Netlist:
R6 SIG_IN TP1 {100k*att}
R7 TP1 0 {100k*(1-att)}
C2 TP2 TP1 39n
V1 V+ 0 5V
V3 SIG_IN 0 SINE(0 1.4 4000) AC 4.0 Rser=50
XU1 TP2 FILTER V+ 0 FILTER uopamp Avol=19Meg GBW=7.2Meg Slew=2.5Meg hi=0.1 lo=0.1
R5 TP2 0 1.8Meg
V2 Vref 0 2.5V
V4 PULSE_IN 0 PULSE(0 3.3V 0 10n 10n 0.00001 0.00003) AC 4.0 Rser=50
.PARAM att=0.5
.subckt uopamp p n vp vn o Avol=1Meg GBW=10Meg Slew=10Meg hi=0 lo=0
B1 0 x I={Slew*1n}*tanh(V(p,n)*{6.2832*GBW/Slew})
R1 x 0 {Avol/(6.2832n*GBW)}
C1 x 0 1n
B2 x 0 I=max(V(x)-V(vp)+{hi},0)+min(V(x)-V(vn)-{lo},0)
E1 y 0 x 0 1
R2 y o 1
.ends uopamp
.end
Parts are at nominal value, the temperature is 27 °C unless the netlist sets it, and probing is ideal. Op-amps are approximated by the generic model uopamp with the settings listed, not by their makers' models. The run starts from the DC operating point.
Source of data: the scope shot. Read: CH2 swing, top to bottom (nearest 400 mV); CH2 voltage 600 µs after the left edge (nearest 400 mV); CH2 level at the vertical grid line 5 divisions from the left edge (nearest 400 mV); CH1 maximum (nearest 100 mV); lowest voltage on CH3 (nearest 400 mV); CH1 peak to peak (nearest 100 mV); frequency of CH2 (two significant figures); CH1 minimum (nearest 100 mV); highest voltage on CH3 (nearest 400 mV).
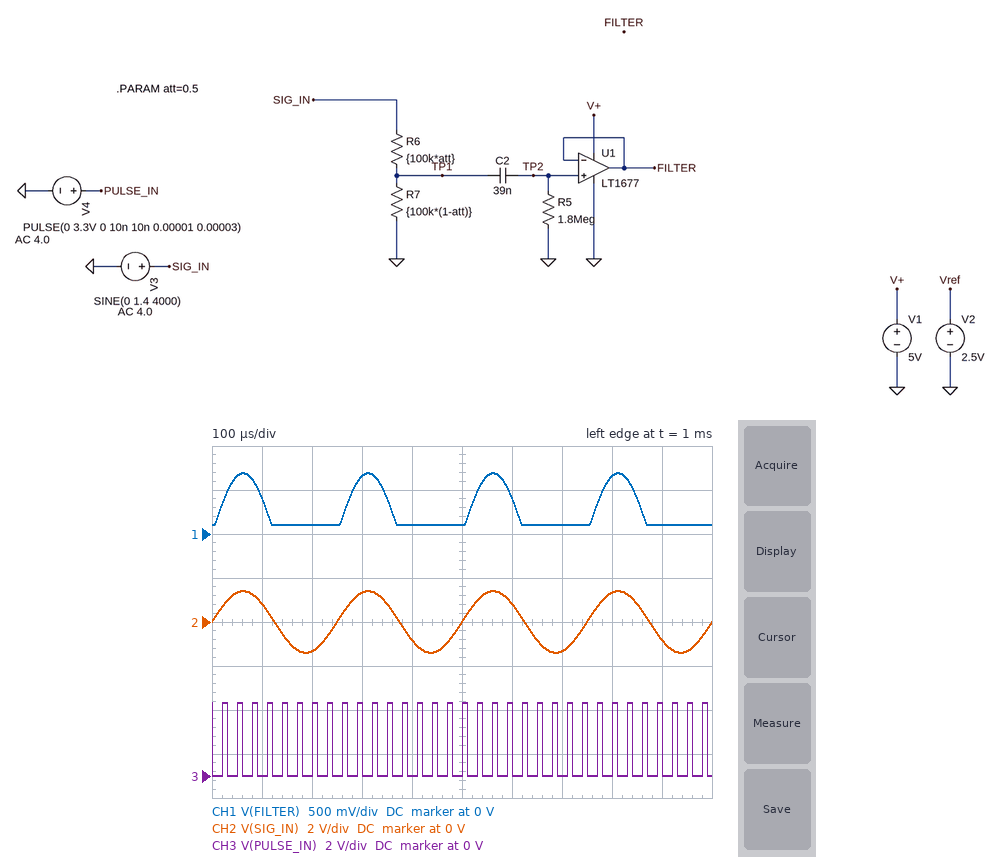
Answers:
2.8 V
800 mV
0 V
700 mV
0 V
600 mV
4.0 kHz
100 mV
3.2 V
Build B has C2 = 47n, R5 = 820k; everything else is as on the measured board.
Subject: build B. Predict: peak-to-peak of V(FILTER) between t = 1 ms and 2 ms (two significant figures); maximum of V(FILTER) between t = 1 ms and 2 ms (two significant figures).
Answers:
580 mV
680 mV
